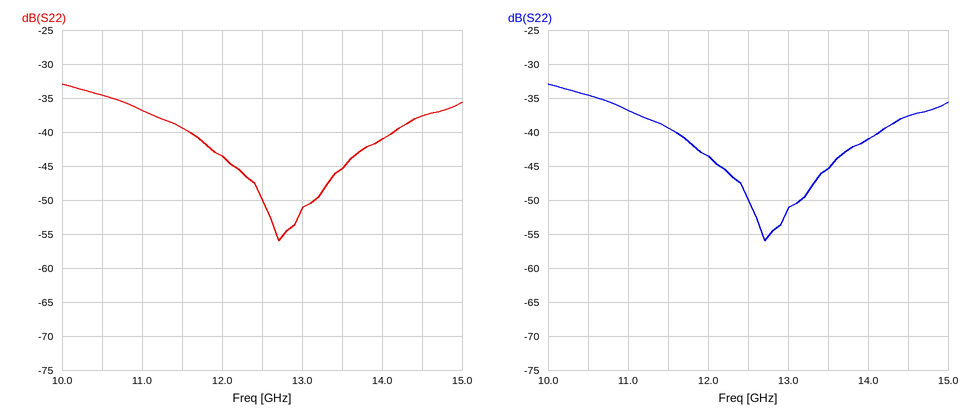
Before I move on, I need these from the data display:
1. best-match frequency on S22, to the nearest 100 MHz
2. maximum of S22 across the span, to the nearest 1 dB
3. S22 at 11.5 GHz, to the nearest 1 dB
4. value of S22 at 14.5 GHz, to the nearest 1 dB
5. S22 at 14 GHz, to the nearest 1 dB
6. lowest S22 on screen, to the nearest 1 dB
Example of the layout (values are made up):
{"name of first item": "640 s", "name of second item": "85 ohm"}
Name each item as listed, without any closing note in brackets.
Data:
{"best-match frequency on S22, to the nearest 100 MHz": "12.7 GHz", "maximum of S22 across the span, to the nearest 1 dB": "-33 dB", "S22 at 11.5 GHz, to the nearest 1 dB": "-39 dB", "value of S22 at 14.5 GHz, to the nearest 1 dB": "-38 dB", "S22 at 14 GHz, to the nearest 1 dB": "-41 dB", "lowest S22 on screen, to the nearest 1 dB": "-56 dB"}
